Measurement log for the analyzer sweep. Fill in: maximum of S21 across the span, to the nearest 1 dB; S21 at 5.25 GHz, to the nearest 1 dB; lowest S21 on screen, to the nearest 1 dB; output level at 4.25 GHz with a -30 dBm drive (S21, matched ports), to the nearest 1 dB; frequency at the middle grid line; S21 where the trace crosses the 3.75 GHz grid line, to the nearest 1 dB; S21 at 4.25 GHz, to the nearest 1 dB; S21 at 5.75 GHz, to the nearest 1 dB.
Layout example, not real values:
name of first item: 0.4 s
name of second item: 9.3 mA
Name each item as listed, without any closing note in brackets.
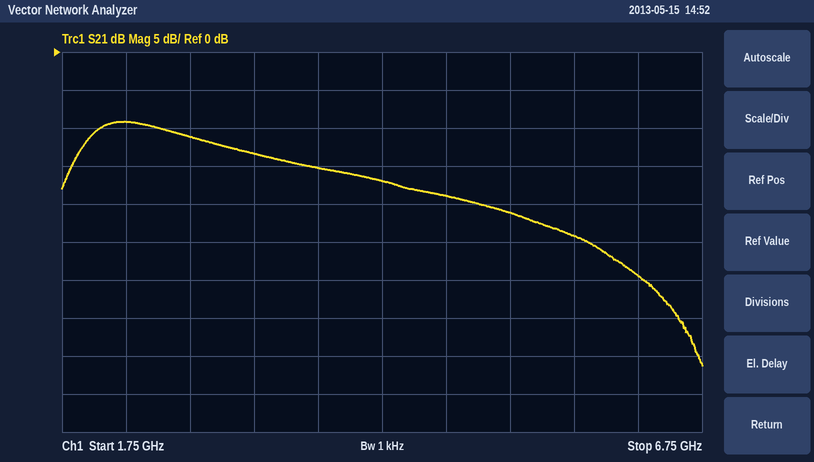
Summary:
maximum of S21 across the span, to the nearest 1 dB: -9 dB
S21 at 5.25 GHz, to the nearest 1 dB: -21 dB
lowest S21 on screen, to the nearest 1 dB: -41 dB
output level at 4.25 GHz with a -30 dBm drive (S21, matched ports), to the nearest 1 dB: -47 dBm
frequency at the middle grid line: 4.25 GHz
S21 where the trace crosses the 3.75 GHz grid line, to the nearest 1 dB: -15 dB
S21 at 4.25 GHz, to the nearest 1 dB: -17 dB
S21 at 5.75 GHz, to the nearest 1 dB: -24 dB
